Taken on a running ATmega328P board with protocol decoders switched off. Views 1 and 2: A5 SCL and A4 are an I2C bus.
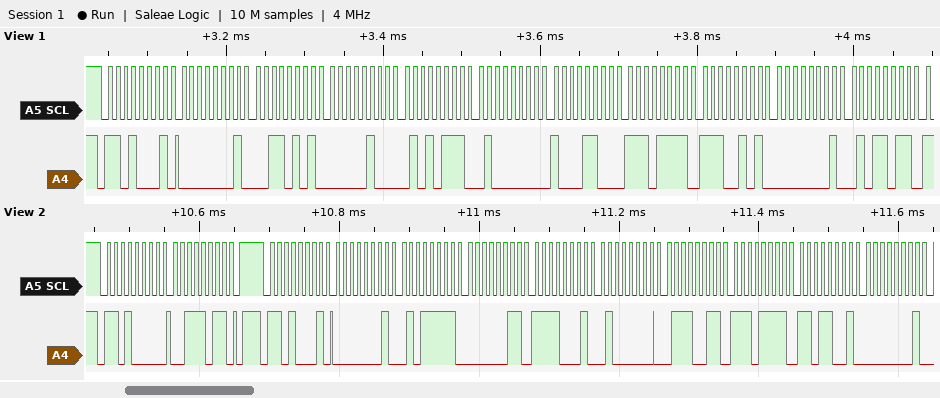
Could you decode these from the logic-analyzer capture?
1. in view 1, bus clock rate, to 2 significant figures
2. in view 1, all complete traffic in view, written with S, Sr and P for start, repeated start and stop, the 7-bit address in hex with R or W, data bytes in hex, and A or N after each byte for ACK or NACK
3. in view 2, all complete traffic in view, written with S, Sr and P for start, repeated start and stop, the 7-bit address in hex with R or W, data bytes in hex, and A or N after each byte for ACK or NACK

100 kHz
S 68R A 01 A 35 A 04 A 57 A 40 A 8C A EF A E5 A 01 A 5B A
S 68W A 3B A P S 68R A 01 A 5F A 03 A F1 A 40 A 73 A EF A D9 A 01 A
